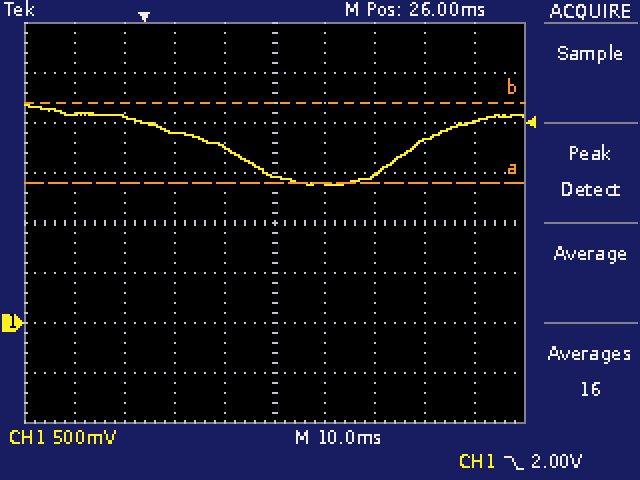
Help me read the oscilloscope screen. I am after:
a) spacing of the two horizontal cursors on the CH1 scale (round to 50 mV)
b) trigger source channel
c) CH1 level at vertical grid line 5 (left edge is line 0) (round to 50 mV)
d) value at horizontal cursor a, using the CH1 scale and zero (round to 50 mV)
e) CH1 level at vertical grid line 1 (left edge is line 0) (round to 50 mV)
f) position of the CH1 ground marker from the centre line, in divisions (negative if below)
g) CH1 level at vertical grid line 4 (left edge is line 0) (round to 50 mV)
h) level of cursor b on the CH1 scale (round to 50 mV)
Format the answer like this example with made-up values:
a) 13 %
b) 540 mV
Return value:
a) 800 mV
b) CH1
c) 1.45 V
d) 1.40 V
e) 2.10 V
f) -2.0 div
g) 1.75 V
h) 2.20 V
